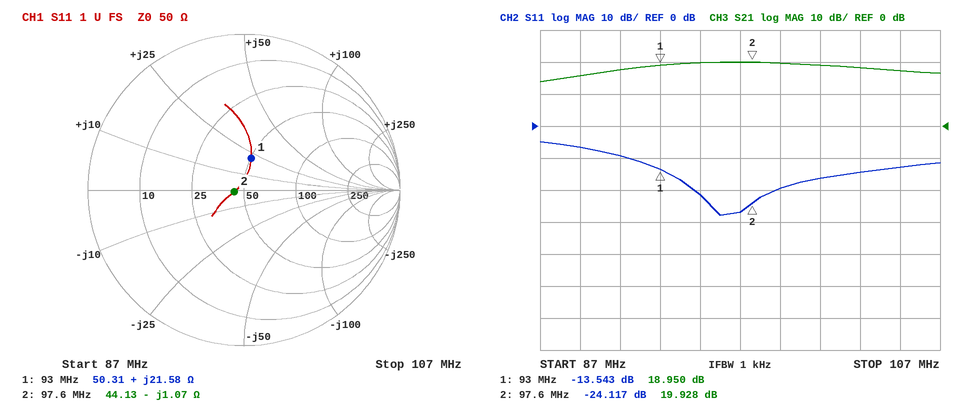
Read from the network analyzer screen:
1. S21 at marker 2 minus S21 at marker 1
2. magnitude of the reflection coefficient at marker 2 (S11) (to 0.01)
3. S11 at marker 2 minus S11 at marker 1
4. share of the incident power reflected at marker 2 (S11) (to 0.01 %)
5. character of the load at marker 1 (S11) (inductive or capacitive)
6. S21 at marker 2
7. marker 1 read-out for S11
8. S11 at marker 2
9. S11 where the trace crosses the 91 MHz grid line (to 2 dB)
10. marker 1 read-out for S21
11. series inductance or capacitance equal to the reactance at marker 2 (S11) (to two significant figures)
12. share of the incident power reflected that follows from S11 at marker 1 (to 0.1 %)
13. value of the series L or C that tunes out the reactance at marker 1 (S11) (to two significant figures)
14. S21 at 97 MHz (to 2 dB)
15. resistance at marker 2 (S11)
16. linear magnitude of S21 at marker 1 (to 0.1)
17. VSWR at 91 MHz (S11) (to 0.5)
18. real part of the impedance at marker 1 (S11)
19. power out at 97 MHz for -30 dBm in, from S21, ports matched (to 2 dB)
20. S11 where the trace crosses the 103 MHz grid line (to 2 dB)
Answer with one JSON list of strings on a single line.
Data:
["0.978 dB", "0.06", "-10.574 dB", "0.39 %", "inductive", "19.928 dB", "-13.543 dB", "-24.117 dB", "-10 dB", "18.950 dB", "1.5 nF", "4.4 %", "79 pF", "20 dB", "44.13 Ω", "8.9", "2.0", "50.31 Ω", "-10 dBm", "-14 dB"]
